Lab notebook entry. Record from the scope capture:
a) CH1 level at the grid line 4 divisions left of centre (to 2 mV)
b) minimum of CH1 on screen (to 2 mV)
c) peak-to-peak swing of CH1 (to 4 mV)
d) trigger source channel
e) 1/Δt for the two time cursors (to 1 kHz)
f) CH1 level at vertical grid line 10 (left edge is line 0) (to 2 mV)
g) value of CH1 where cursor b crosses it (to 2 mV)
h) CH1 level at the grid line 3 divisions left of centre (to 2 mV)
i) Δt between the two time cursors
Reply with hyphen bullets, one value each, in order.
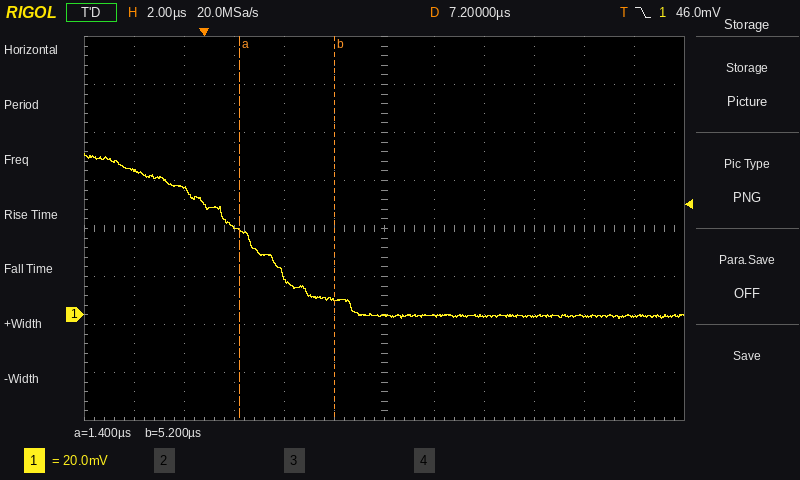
- 52 mV
- -2 mV
- 68 mV
- CH1
- 263 kHz
- 0 mV
- 6 mV
- 36 mV
- 3.8 µs
